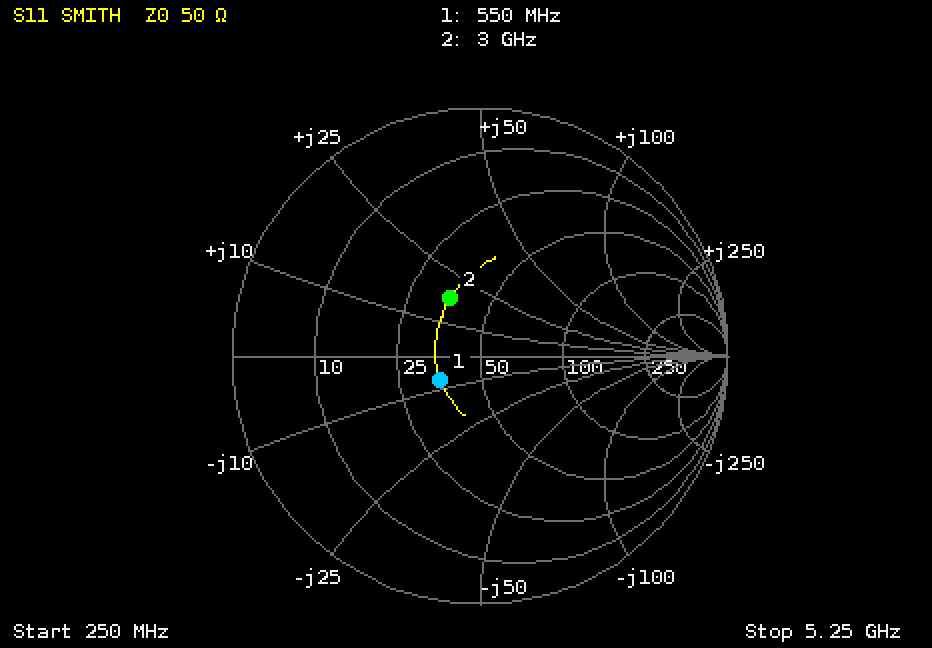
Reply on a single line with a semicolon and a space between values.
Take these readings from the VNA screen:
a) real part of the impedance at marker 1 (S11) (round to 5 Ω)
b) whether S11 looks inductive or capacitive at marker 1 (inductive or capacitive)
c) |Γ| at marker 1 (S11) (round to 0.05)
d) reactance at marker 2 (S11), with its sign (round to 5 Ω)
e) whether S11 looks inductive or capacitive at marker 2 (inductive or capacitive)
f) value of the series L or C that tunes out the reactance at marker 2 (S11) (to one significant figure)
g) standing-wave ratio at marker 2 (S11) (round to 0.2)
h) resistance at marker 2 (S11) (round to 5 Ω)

35 Ω; capacitive; 0.20; +20 Ω; inductive; 3 pF; 1.8; 35 Ω
